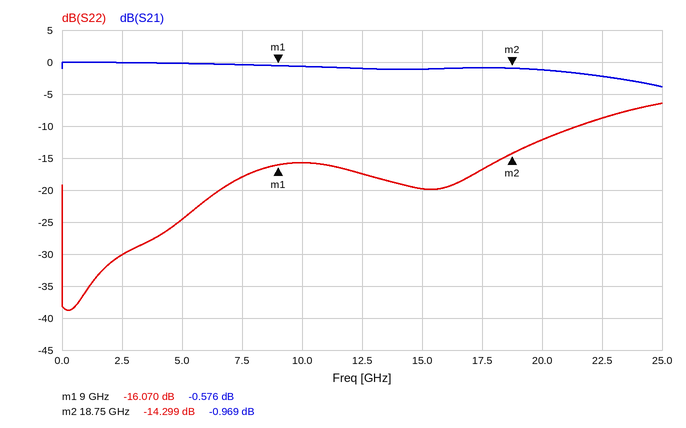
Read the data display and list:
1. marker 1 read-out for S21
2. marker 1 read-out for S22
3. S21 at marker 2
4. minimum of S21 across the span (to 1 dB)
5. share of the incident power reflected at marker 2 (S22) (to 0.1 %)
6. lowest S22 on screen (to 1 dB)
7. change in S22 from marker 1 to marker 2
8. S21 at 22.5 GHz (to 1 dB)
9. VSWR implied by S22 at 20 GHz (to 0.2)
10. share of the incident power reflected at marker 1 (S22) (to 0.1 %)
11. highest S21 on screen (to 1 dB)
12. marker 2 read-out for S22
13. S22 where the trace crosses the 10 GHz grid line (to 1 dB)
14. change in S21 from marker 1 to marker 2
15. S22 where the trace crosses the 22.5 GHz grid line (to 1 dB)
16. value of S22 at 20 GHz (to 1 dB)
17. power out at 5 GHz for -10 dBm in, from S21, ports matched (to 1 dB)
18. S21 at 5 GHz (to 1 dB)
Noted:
-0.576 dB
-16.070 dB
-0.969 dB
-4 dB
3.7 %
-39 dB
1.771 dB
-2 dB
1.6
2.5 %
0 dB
-14.299 dB
-16 dB
-0.393 dB
-9 dB
-12 dB
-10 dBm
0 dB
